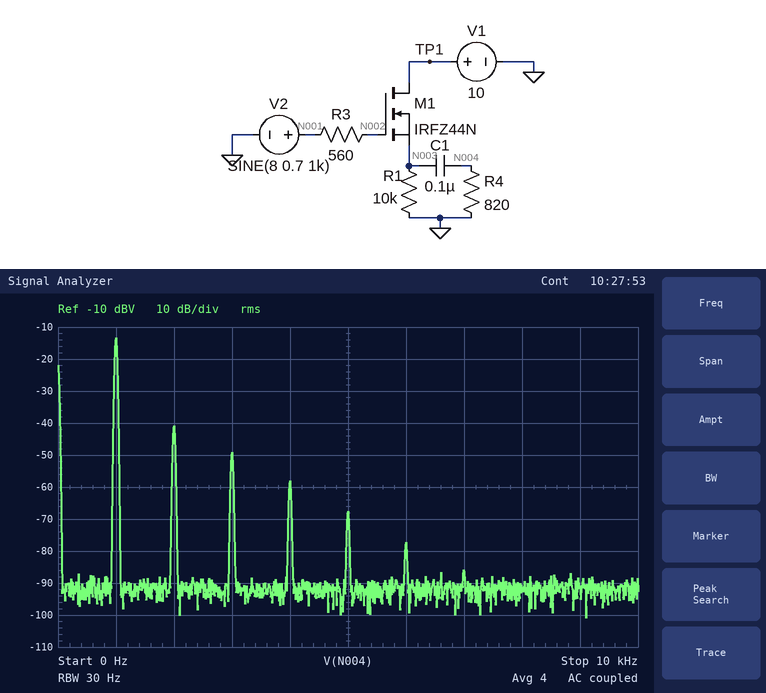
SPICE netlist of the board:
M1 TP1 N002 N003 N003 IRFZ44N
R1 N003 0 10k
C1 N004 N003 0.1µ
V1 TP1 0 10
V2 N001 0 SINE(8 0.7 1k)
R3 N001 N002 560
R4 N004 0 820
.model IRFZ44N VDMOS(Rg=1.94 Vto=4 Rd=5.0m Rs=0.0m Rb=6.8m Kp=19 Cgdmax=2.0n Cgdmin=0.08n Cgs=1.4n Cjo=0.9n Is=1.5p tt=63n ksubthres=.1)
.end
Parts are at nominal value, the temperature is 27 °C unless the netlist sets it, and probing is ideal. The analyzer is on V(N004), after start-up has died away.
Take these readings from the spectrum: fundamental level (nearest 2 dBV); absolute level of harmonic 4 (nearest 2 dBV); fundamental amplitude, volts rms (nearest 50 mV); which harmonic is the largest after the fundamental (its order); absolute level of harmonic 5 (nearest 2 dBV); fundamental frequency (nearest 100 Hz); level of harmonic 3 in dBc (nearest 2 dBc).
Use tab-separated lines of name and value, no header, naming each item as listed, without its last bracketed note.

fundamental level	-14 dBV
absolute level of harmonic 4	-58 dBV
fundamental amplitude, volts rms	200 mV
which harmonic is the largest after the fundamental	2
absolute level of harmonic 5	-68 dBV
fundamental frequency	1.0 kHz
level of harmonic 3 in dBc	-36 dBc
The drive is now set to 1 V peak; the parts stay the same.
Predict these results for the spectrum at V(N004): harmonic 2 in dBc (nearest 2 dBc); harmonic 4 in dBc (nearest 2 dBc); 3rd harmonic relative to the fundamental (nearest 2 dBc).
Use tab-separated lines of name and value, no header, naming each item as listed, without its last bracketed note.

harmonic 2 in dBc	-18 dBc
harmonic 4 in dBc	-32 dBc
3rd harmonic relative to the fundamental	-24 dBc
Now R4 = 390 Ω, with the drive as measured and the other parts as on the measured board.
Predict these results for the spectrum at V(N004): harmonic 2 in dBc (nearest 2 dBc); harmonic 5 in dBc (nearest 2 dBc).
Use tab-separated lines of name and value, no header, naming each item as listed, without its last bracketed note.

harmonic 2 in dBc	-24 dBc
harmonic 5 in dBc	-48 dBc
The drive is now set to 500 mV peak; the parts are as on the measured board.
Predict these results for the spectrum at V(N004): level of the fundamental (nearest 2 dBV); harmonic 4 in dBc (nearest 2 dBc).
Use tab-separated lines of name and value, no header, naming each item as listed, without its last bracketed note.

level of the fundamental	-16 dBV
harmonic 4 in dBc	-58 dBc
